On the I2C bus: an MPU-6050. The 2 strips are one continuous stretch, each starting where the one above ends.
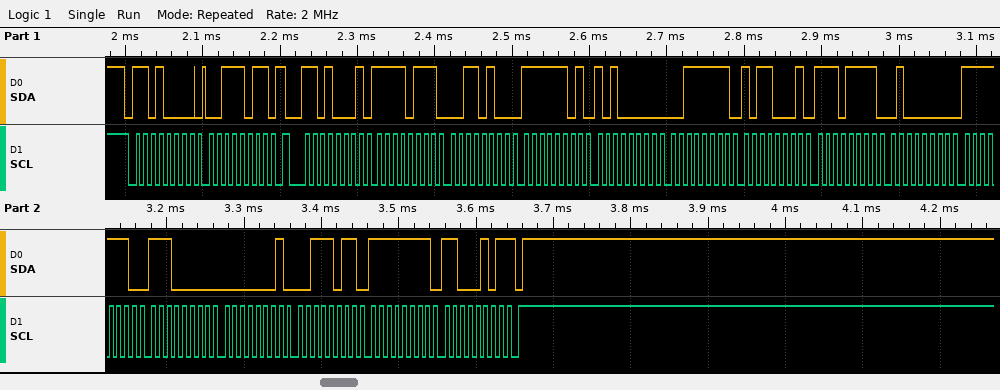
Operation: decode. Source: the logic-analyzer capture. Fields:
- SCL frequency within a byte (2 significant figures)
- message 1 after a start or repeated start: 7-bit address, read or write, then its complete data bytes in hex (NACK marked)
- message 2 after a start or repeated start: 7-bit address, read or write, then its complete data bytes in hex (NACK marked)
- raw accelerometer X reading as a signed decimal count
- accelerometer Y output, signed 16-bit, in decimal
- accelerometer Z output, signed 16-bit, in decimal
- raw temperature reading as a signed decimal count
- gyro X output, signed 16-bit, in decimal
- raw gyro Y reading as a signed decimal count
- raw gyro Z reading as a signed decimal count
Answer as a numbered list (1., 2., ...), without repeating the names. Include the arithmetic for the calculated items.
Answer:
1. 100 kHz
2. 0x68 write: 3B
3. 0x68 read: F7 34 FD A0 3F B1 EF 40 FE E0 01 3B FF C5 NACK
4. 0xF734 = -2252
5. 0xFDA0 = -608
6. 0x3FB1 = 16305
7. 0xEF40 = -4288
8. 0xFEE0 = -288
9. 0x013B = 315
10. 0xFFC5 = -59
